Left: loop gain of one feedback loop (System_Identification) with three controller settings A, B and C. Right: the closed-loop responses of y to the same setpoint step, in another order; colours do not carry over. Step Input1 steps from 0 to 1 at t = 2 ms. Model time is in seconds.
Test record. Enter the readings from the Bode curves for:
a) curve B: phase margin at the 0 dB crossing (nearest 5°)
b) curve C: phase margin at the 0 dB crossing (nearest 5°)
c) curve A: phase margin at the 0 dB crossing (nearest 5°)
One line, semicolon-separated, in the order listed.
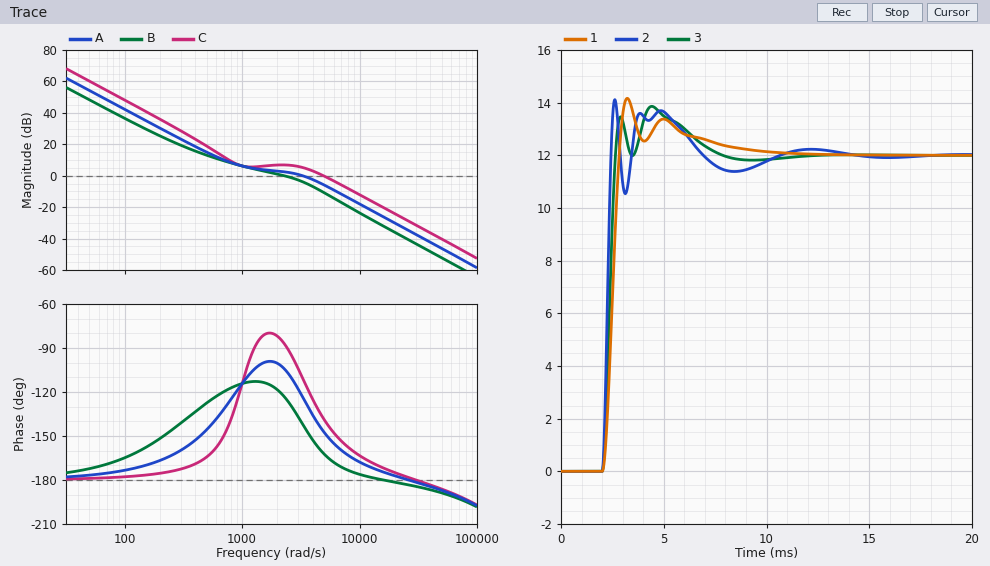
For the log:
55°; 40°; 55°
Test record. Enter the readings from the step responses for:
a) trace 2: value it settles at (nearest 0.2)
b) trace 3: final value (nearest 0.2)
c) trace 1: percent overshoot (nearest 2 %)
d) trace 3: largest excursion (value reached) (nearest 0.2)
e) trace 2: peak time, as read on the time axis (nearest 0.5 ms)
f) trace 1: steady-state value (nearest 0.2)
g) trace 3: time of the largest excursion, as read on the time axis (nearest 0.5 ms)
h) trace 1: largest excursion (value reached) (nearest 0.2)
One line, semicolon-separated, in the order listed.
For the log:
12.0; 12.0; 18 %; 13.8; 2.5 ms; 12.0; 4.5 ms; 14.2
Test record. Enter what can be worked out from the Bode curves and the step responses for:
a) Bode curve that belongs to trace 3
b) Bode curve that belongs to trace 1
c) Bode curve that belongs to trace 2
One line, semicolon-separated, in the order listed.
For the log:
A; B; C
